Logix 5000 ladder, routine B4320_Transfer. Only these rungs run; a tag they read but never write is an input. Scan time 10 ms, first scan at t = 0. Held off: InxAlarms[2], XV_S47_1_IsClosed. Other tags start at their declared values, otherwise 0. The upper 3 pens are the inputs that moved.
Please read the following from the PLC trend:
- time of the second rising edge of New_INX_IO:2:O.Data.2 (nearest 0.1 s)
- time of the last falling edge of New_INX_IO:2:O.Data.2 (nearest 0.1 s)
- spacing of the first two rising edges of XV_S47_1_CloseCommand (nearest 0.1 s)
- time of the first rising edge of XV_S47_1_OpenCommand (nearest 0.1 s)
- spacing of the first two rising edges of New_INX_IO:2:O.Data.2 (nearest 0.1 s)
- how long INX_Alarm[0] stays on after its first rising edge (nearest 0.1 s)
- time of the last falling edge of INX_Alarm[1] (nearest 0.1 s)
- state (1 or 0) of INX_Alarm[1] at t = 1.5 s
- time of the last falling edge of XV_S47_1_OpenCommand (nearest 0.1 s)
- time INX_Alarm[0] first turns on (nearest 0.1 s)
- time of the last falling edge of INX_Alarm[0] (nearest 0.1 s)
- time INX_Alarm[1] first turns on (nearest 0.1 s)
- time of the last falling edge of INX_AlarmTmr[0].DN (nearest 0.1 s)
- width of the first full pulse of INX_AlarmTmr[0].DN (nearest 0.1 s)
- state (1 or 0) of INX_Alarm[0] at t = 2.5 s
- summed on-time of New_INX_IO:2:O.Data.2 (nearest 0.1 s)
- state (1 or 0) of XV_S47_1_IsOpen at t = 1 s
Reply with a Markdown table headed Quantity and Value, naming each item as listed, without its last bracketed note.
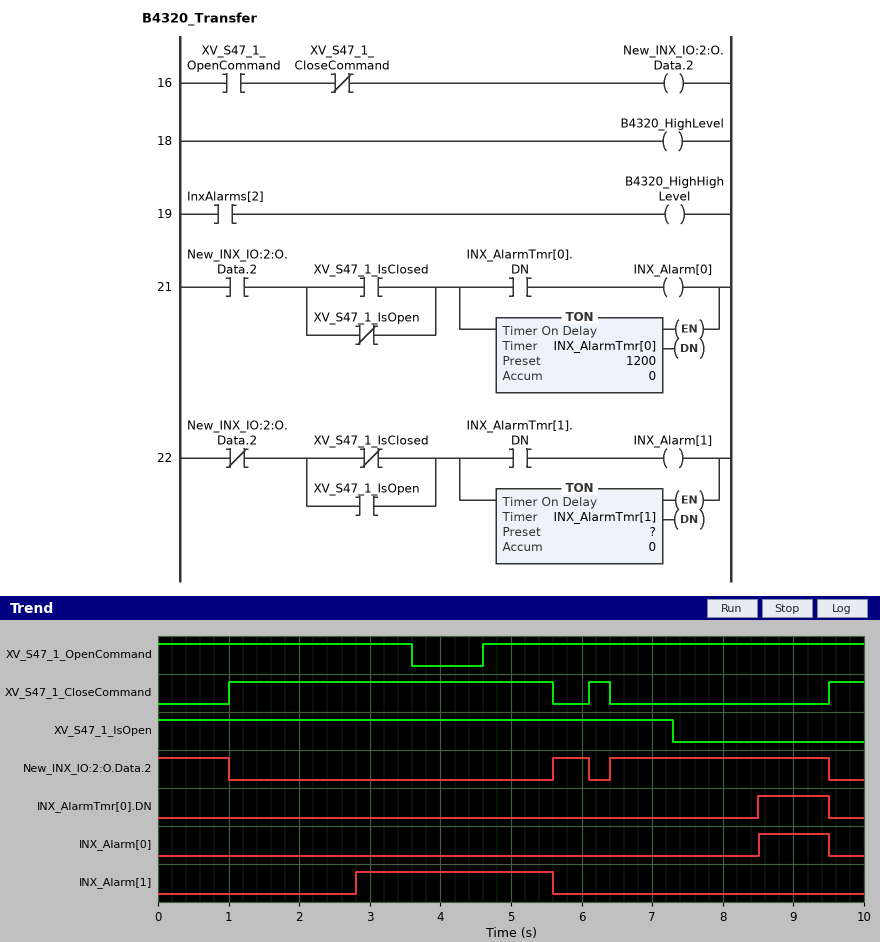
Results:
| Quantity | Value |
|---|---|
| time of the second rising edge of New_INX_IO:2:O.Data.2 | 6.4 s |
| time of the last falling edge of New_INX_IO:2:O.Data.2 | 9.5 s |
| spacing of the first two rising edges of XV_S47_1_CloseCommand | 5.1 s |
| time of the first rising edge of XV_S47_1_OpenCommand | 4.6 s |
| spacing of the first two rising edges of New_INX_IO:2:O.Data.2 | 0.8 s |
| how long INX_Alarm[0] stays on after its first rising edge | 1.0 s |
| time of the last falling edge of INX_Alarm[1] | 5.6 s |
| state (1 or 0) of INX_Alarm[1] at t = 1.5 s | 0 |
| time of the last falling edge of XV_S47_1_OpenCommand | 3.6 s |
| time INX_Alarm[0] first turns on | 8.5 s |
| time of the last falling edge of INX_Alarm[0] | 9.5 s |
| time INX_Alarm[1] first turns on | 2.8 s |
| time of the last falling edge of INX_AlarmTmr[0].DN | 9.5 s |
| width of the first full pulse of INX_AlarmTmr[0].DN | 1.0 s |
| state (1 or 0) of INX_Alarm[0] at t = 2.5 s | 0 |
| summed on-time of New_INX_IO:2:O.Data.2 | 4.6 s |
| state (1 or 0) of XV_S47_1_IsOpen at t = 1 s | 1 |
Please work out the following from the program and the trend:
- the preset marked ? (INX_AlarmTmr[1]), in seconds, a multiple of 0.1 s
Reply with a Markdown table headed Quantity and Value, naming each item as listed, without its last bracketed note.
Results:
| Quantity | Value |
|---|---|
| the preset marked ? (INX_AlarmTmr[1]), in seconds, a multiple of 0.1 s | 1.8 s |
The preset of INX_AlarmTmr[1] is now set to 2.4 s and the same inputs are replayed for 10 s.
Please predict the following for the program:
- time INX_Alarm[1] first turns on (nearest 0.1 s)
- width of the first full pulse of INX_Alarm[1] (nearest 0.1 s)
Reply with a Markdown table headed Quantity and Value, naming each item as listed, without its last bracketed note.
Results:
| Quantity | Value |
|---|---|
| time INX_Alarm[1] first turns on | 3.4 s |
| width of the first full pulse of INX_Alarm[1] | 2.2 s |
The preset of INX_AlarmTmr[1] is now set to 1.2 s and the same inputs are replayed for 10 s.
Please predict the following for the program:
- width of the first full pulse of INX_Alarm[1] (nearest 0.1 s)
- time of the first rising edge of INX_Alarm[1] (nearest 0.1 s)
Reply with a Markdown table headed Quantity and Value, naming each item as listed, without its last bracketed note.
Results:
| Quantity | Value |
|---|---|
| width of the first full pulse of INX_Alarm[1] | 3.4 s |
| time of the first rising edge of INX_Alarm[1] | 2.2 s |
